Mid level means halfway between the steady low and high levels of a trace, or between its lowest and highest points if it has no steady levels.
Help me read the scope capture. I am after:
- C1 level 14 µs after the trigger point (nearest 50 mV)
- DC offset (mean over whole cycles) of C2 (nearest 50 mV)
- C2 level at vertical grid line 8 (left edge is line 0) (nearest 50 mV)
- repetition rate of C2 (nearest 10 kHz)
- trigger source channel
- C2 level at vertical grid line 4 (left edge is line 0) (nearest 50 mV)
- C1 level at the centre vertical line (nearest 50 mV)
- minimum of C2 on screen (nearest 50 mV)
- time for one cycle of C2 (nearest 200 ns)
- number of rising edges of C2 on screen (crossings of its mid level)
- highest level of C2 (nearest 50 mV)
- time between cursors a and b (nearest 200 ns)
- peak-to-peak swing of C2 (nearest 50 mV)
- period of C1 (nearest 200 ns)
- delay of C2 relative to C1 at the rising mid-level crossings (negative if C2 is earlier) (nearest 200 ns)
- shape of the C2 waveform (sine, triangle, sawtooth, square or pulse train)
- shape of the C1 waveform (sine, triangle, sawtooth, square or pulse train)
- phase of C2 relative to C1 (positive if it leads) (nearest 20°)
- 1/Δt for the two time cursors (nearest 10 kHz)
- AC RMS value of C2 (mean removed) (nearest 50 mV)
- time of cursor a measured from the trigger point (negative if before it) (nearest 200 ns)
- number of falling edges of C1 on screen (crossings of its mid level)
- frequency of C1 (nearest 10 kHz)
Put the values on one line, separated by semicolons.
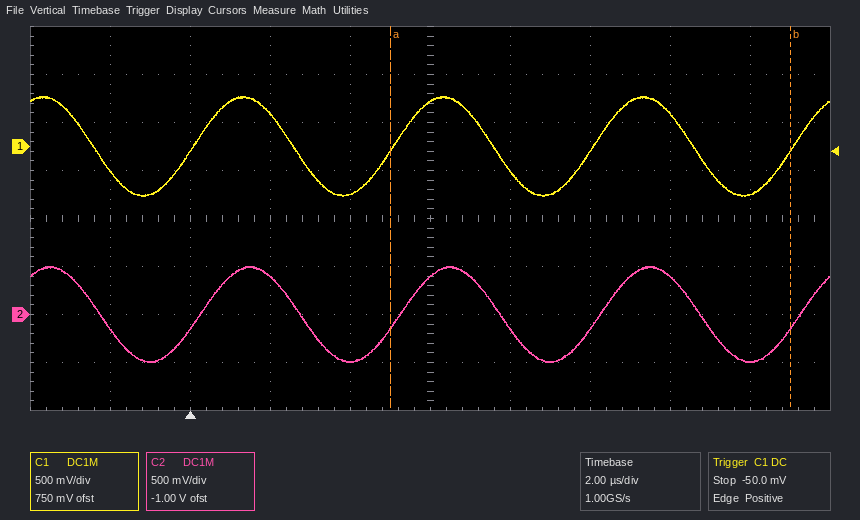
-500 mV; 0 mV; 400 mV; 200 kHz; C1; -500 mV; 450 mV; -500 mV; 5.0 µs; 4; 500 mV; 10.0 µs; 1.00 V; 5.0 µs; +200 ns; sine; sine; -20°; 100 kHz; 350 mV; +5.0 µs; 4; 200 kHz
